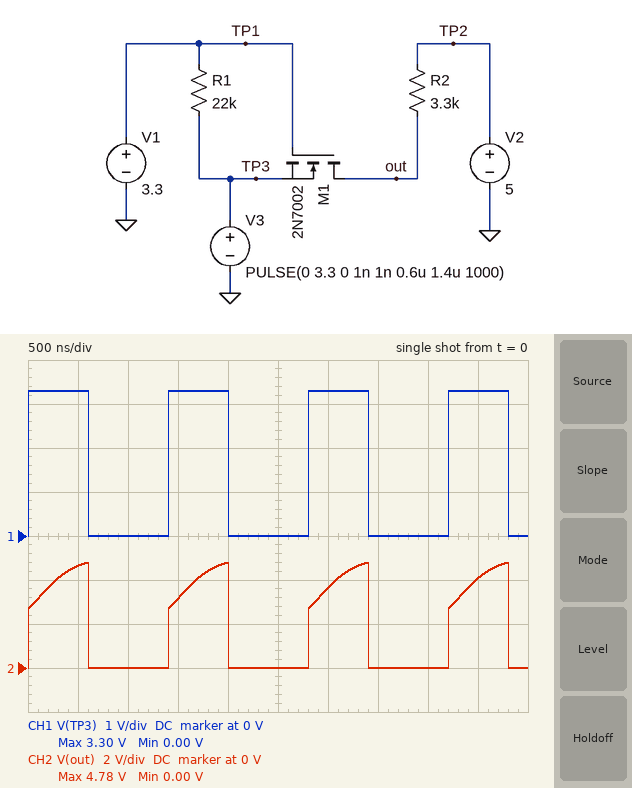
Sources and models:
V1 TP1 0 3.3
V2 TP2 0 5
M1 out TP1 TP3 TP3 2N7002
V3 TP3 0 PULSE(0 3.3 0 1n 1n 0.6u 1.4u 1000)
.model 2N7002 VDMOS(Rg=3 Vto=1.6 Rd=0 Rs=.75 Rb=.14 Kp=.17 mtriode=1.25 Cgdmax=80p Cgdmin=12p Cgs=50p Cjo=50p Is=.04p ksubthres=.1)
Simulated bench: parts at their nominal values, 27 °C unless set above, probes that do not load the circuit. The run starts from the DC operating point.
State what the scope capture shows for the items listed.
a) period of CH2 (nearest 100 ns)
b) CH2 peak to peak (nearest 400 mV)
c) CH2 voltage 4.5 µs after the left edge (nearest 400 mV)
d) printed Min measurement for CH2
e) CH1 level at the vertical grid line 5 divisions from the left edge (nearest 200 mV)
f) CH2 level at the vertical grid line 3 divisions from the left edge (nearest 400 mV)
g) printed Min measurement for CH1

1.4 µs
4.8 V
4.0 V
0.00 V
0 V
3.2 V
0.00 V
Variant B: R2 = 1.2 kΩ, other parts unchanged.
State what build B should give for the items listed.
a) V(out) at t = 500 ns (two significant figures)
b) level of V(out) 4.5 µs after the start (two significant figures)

5.0 V
4.9 V
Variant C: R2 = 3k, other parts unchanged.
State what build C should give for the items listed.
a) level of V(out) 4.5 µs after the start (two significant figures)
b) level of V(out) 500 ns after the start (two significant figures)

4.2 V
4.7 V
